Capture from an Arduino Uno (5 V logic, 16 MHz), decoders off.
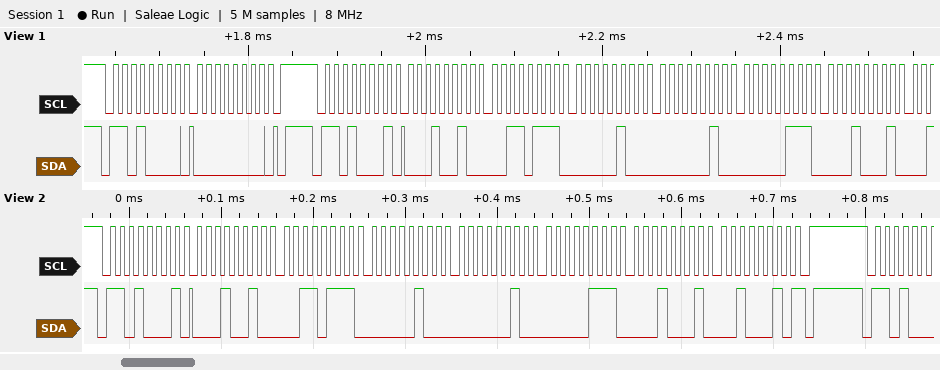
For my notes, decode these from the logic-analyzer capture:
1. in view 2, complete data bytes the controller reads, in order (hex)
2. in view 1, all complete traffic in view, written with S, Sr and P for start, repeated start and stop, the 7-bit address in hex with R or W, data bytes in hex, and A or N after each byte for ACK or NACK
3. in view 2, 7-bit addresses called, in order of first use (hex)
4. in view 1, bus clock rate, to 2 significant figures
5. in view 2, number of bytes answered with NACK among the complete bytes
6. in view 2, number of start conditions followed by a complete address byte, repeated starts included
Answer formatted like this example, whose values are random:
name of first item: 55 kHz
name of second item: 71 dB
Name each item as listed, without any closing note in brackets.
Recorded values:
in view 2, complete data bytes the controller reads, in order: 12 37 04 02 07 11 22
in view 1, all complete traffic in view, written with S, Sr and P for start, repeated start and stop, the 7-bit address in hex with R or W, data bytes in hex, and A or N after each byte for ACK or NACK: S 68W A 00 A P S 68R A 12 A 37 A 04 A 02 A 07 A 11 A
in view 2, 7-bit addresses called, in order of first use: 0x68
in view 1, bus clock rate, to 2 significant figures: 100 kHz
in view 2, number of bytes answered with NACK among the complete bytes: 1
in view 2, number of start conditions followed by a complete address byte, repeated starts included: 1
